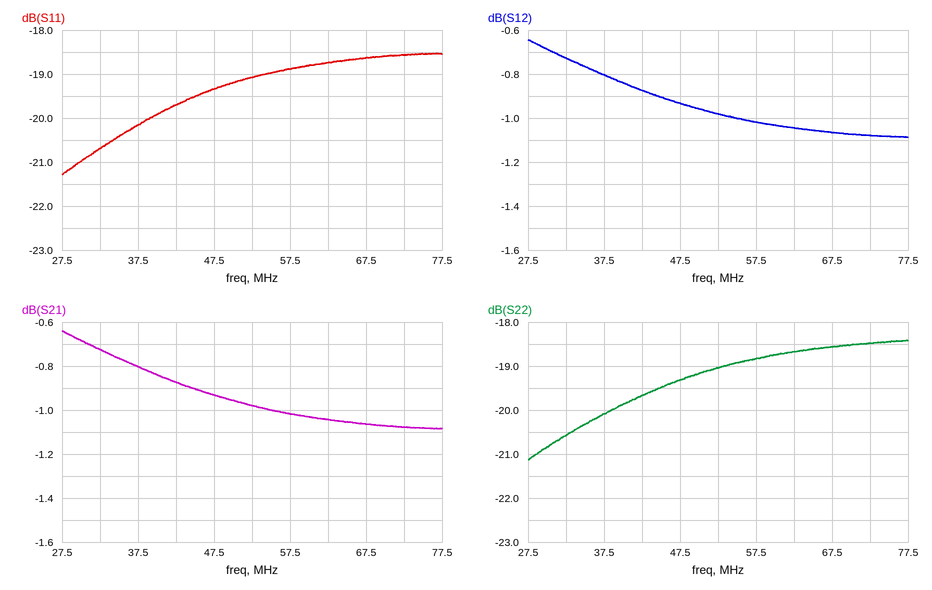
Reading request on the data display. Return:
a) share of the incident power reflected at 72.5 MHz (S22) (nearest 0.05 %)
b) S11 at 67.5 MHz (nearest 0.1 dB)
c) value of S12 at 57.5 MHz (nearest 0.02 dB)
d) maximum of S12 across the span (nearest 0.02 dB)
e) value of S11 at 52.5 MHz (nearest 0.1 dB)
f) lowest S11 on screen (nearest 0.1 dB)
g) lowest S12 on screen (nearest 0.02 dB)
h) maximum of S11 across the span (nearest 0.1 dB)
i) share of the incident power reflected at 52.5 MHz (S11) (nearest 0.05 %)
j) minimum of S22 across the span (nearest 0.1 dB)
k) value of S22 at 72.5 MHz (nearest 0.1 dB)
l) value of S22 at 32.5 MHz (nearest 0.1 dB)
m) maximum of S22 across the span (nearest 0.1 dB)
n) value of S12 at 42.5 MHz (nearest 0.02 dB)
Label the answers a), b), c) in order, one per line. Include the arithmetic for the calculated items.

a) 10^(-18.5/10) ≈ 1.41 %, so 1.40 % to the nearest 0.05 %
b) -18.6 dB
c) -1.02 dB
d) -0.64 dB
e) -19.1 dB
f) -21.3 dB
g) -1.08 dB
h) -18.5 dB
i) 10^(-19.1/10) ≈ 1.23 %, so 1.25 % to the nearest 0.05 %
j) -21.1 dB
k) -18.5 dB
l) -20.6 dB
m) -18.4 dB
n) -0.88 dB
